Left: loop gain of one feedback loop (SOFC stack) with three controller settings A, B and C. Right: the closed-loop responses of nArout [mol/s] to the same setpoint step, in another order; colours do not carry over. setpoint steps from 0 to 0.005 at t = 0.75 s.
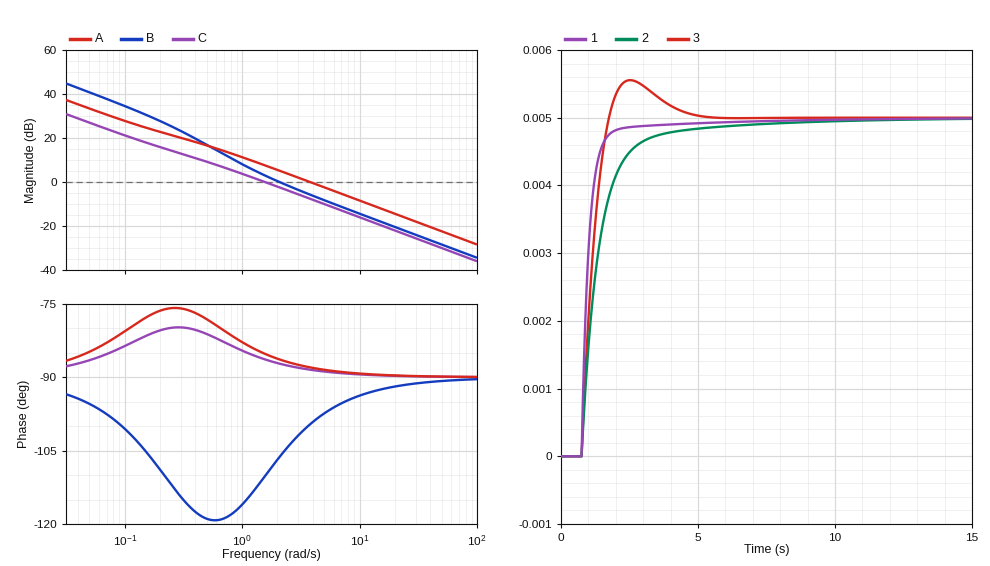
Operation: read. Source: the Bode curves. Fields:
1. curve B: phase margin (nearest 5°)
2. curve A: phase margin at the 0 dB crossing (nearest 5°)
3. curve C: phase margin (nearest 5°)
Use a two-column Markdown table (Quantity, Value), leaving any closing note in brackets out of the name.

| Quantity | Value |
|---|---|
| curve B: phase margin | 75° |
| curve A: phase margin at the 0 dB crossing | 90° |
| curve C: phase margin | 95° |
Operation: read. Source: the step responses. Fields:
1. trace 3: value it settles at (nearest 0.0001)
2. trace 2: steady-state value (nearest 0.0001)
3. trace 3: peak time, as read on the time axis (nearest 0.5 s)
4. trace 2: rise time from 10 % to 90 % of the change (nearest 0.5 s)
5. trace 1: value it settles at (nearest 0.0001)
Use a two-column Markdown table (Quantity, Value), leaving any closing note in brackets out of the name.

| Quantity | Value |
|---|---|
| trace 3: value it settles at | 0.0050 |
| trace 2: steady-state value | 0.0050 |
| trace 3: peak time, as read on the time axis | 2.5 s |
| trace 2: rise time from 10 % to 90 % of the change | 1.5 s |
| trace 1: value it settles at | 0.0050 |
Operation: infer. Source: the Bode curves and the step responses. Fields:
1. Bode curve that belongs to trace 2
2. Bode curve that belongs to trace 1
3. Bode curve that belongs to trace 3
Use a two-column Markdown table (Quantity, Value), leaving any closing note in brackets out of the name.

| Quantity | Value |
|---|---|
| Bode curve that belongs to trace 2 | C |
| Bode curve that belongs to trace 1 | A |
| Bode curve that belongs to trace 3 | B |
